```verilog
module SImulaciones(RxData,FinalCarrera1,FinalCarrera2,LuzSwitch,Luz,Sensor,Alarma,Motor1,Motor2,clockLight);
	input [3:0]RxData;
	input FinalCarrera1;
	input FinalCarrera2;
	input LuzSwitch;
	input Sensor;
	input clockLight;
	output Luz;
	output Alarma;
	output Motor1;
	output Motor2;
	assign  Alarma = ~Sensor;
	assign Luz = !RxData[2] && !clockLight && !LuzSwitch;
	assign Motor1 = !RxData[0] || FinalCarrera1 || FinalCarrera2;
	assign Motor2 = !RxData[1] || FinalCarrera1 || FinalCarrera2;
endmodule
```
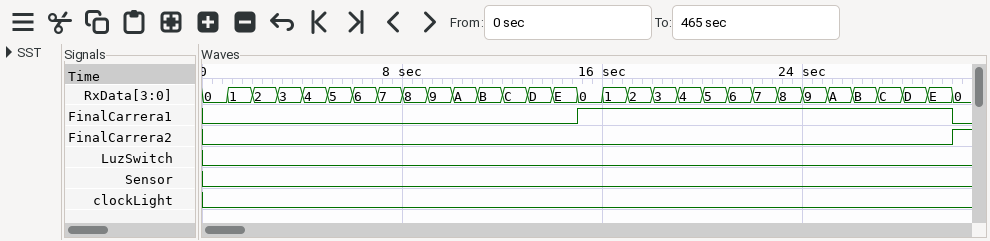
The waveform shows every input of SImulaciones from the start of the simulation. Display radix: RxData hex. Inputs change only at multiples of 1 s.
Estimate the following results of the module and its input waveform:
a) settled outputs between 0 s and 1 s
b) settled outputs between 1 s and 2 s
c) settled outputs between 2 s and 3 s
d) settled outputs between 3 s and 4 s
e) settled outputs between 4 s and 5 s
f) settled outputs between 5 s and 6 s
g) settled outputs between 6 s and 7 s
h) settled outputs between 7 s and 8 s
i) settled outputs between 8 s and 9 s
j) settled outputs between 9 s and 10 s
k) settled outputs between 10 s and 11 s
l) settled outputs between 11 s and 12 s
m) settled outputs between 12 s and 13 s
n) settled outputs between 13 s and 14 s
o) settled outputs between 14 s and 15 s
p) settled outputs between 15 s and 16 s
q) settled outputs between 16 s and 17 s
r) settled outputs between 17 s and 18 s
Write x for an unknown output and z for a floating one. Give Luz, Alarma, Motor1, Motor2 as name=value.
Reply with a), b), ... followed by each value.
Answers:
a) Luz=1, Alarma=1, Motor1=1, Motor2=1
b) Luz=1, Alarma=1, Motor1=0, Motor2=1
c) Luz=1, Alarma=1, Motor1=1, Motor2=0
d) Luz=1, Alarma=1, Motor1=0, Motor2=0
e) Luz=0, Alarma=1, Motor1=1, Motor2=1
f) Luz=0, Alarma=1, Motor1=0, Motor2=1
g) Luz=0, Alarma=1, Motor1=1, Motor2=0
h) Luz=0, Alarma=1, Motor1=0, Motor2=0
i) Luz=1, Alarma=1, Motor1=1, Motor2=1
j) Luz=1, Alarma=1, Motor1=0, Motor2=1
k) Luz=1, Alarma=1, Motor1=1, Motor2=0
l) Luz=1, Alarma=1, Motor1=0, Motor2=0
m) Luz=0, Alarma=1, Motor1=1, Motor2=1
n) Luz=0, Alarma=1, Motor1=0, Motor2=1
o) Luz=0, Alarma=1, Motor1=1, Motor2=0
p) Luz=1, Alarma=1, Motor1=1, Motor2=1
q) Luz=1, Alarma=1, Motor1=1, Motor2=1
r) Luz=1, Alarma=1, Motor1=1, Motor2=1
